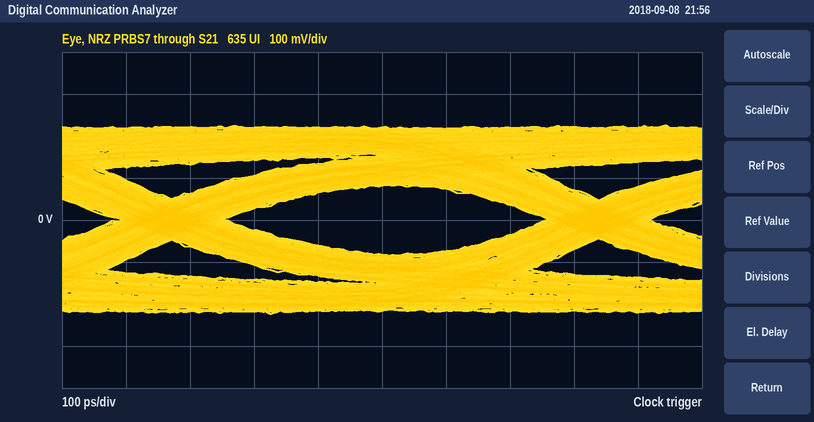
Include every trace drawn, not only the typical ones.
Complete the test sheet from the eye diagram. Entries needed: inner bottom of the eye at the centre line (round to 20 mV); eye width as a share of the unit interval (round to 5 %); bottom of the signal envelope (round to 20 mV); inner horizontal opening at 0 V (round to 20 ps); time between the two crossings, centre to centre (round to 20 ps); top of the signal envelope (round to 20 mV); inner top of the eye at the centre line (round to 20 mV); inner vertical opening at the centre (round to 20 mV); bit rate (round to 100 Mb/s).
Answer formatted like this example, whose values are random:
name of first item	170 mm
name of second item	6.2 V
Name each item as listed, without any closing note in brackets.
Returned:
inner bottom of the eye at the centre line	-80 mV
eye width as a share of the unit interval	75 %
bottom of the signal envelope	-220 mV
inner horizontal opening at 0 V	500 ps
time between the two crossings, centre to centre	660 ps
top of the signal envelope	220 mV
inner top of the eye at the centre line	80 mV
inner vertical opening at the centre	160 mV
bit rate	1.5 Gb/s
